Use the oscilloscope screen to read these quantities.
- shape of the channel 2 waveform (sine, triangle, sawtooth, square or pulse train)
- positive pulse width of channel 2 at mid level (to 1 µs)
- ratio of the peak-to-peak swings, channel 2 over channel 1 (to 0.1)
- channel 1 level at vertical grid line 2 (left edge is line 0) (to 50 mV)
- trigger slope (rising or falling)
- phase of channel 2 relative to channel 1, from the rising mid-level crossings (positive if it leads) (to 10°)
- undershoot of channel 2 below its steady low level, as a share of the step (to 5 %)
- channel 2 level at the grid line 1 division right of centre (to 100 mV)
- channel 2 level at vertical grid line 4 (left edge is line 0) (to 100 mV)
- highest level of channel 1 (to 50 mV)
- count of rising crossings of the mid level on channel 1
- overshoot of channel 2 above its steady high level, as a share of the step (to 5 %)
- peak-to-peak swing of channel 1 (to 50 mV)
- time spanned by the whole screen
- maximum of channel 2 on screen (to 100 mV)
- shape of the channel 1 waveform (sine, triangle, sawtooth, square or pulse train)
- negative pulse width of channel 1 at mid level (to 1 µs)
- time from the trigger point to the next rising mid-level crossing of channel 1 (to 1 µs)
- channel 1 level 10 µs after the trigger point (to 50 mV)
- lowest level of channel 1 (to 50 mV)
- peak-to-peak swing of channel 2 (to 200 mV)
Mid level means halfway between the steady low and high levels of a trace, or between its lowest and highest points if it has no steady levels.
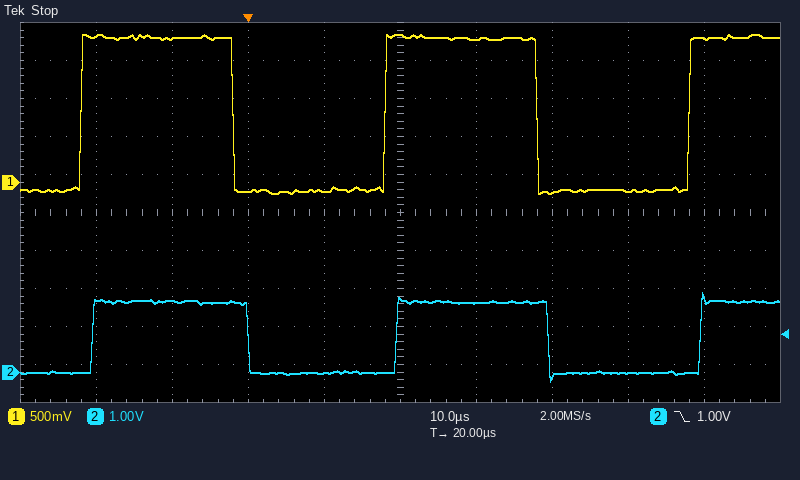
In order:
square
20 µs
1.1
1.90 V
falling
-10°
15 %
1.8 V
0.0 V
1.95 V
3
15 %
2.10 V
100 µs
2.1 V
square
20 µs
18 µs
-100 mV
-150 mV
2.4 V
